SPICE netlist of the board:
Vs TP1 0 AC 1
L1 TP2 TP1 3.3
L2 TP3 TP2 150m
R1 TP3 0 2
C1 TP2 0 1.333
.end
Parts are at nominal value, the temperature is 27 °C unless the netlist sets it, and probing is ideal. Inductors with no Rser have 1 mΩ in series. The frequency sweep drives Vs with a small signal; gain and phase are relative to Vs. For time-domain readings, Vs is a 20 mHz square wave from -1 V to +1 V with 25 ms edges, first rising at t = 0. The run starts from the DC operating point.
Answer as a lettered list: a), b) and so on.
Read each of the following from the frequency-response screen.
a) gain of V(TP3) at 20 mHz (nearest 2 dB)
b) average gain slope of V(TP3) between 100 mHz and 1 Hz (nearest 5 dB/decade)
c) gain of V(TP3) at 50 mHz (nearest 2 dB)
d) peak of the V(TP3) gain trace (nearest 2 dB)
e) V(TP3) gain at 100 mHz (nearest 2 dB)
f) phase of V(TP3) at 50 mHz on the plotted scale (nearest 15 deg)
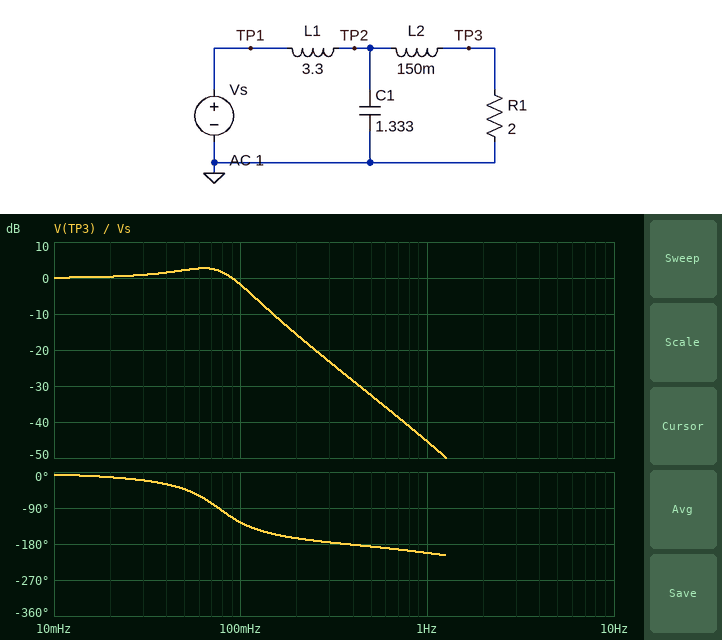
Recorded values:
a) 0 dB
b) -45 dB/decade
c) 2 dB
d) 2 dB
e) -2 dB
f) -45 deg
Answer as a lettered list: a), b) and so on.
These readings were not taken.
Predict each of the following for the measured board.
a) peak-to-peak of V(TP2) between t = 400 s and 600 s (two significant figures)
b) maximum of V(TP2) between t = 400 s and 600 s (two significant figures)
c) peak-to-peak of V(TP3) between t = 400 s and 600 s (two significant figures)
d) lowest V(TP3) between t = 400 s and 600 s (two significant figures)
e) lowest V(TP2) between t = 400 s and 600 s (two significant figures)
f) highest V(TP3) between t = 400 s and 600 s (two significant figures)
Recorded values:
a) 3.0 V
b) 1.5 V
c) 3.0 V
d) -1.5 V
e) -1.5 V
f) 1.5 V
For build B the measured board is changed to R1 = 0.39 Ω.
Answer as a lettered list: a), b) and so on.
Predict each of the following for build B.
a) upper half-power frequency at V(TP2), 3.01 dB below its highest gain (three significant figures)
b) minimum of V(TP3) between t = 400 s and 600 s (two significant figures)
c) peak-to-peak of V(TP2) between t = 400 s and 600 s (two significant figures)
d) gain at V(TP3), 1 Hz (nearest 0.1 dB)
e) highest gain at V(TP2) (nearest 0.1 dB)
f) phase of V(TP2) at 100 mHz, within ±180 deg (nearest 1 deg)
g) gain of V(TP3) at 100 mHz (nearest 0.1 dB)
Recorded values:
a) 19.3 mHz
b) -900 mV
c) 1.8 V
d) -52.1 dB
e) 0 dB
f) -85 deg
g) -14.3 dB
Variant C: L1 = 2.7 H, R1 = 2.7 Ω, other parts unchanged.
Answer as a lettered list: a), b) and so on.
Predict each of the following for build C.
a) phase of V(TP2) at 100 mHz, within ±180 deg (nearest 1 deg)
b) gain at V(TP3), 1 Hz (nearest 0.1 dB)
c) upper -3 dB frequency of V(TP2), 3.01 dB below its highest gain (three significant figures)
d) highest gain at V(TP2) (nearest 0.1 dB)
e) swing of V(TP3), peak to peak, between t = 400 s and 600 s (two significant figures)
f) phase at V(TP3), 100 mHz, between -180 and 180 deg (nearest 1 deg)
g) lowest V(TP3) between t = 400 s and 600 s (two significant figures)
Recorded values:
a) -122 deg
b) -43.4 dB
c) 99.0 mHz
d) 5.8 dB
e) 3.6 V
f) -124 deg
g) -1.8 V
